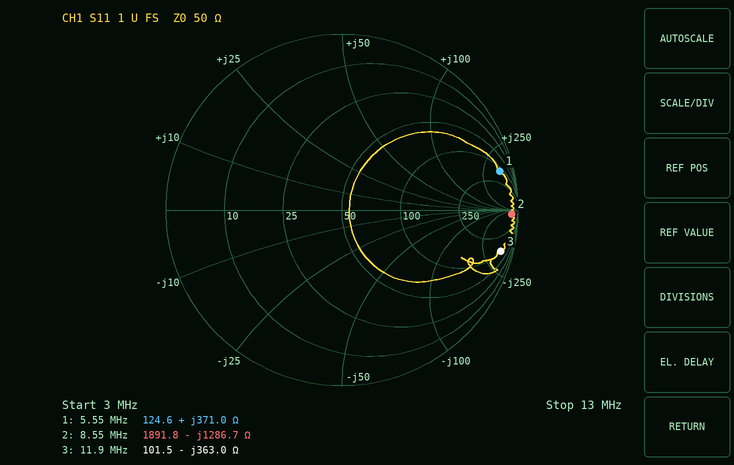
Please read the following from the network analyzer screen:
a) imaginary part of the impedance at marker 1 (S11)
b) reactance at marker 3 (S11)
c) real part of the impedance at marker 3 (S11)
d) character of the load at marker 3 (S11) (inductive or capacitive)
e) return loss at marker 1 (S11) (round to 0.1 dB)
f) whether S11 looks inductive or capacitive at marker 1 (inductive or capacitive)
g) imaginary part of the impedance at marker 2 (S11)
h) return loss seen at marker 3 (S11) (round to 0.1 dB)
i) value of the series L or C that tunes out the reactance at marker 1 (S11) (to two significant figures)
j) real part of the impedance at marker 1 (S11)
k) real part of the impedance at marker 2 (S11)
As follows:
+371.0 Ω
-363.0 Ω
101.5 Ω
capacitive
0.7 dB
inductive
-1286.7 Ω
0.6 dB
77 pF
124.6 Ω
1891.8 Ω
